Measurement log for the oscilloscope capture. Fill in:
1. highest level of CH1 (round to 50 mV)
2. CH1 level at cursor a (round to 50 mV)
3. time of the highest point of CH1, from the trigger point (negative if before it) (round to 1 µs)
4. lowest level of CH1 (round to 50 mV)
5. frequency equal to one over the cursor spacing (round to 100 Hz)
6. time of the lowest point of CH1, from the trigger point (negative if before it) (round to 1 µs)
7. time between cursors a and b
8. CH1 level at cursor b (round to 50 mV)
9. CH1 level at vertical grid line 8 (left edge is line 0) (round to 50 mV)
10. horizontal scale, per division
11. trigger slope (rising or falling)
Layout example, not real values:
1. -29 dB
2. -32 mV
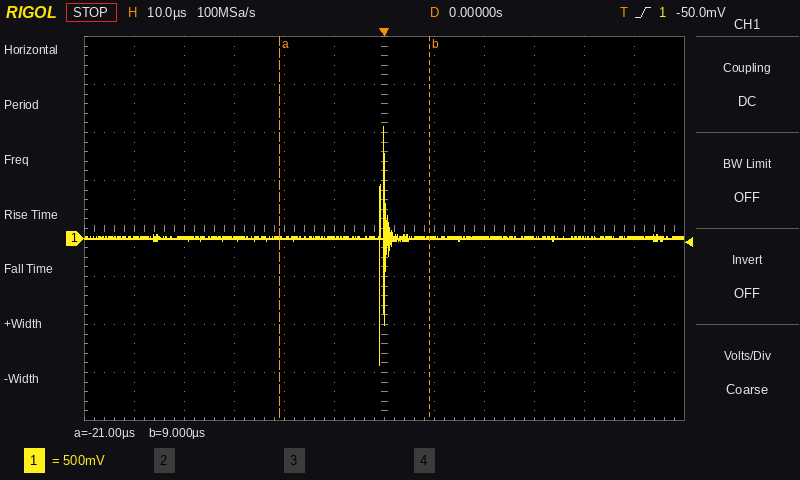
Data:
1. 1.15 V
2. 0 mV
3. 0 µs
4. -1.30 V
5. 33.3 kHz
6. -1 µs
7. 30 µs
8. 0 mV
9. 0 mV
10. 10 µs
11. rising
